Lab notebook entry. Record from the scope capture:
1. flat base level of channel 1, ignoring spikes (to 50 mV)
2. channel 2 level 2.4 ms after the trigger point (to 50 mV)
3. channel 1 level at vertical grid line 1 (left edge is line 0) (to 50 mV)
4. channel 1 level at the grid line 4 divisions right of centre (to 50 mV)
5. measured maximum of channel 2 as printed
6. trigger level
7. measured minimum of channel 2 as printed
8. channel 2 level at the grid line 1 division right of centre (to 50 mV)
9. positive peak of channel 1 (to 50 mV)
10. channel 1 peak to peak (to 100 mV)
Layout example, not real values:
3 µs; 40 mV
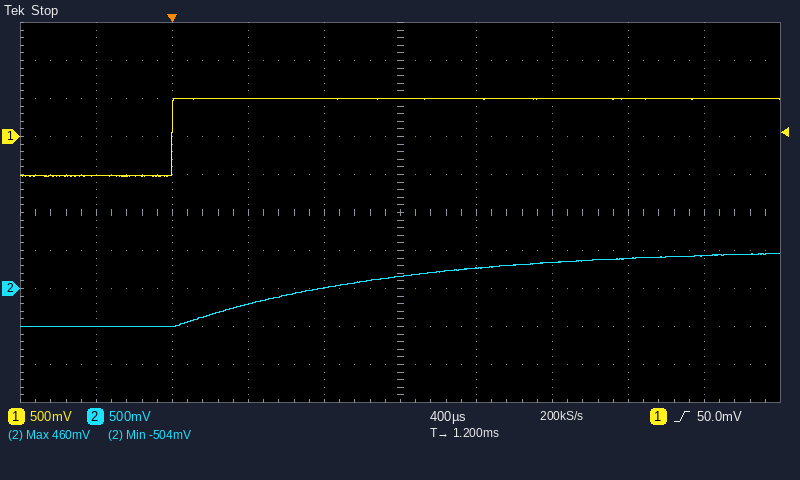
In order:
-500 mV; 400 mV; -500 mV; 500 mV; 460 mV; 50.0 mV; -504 mV; 250 mV; 500 mV; 1.00 V
